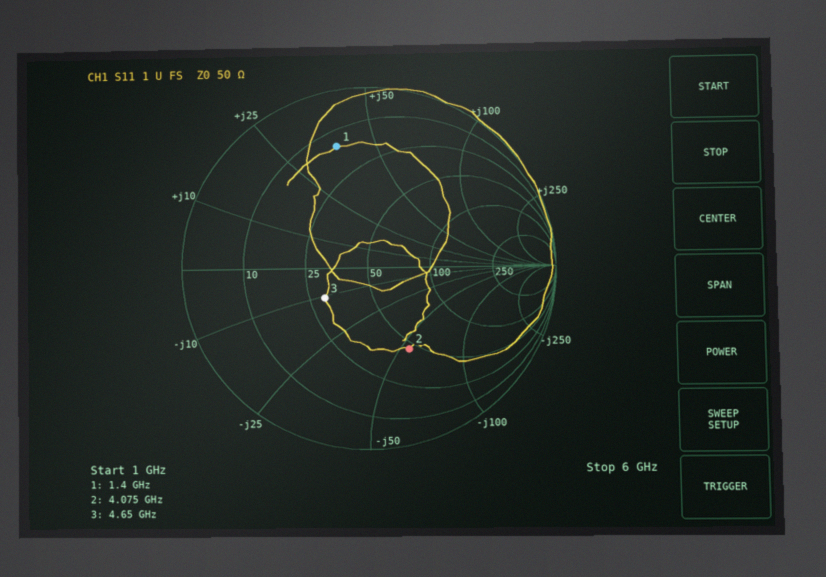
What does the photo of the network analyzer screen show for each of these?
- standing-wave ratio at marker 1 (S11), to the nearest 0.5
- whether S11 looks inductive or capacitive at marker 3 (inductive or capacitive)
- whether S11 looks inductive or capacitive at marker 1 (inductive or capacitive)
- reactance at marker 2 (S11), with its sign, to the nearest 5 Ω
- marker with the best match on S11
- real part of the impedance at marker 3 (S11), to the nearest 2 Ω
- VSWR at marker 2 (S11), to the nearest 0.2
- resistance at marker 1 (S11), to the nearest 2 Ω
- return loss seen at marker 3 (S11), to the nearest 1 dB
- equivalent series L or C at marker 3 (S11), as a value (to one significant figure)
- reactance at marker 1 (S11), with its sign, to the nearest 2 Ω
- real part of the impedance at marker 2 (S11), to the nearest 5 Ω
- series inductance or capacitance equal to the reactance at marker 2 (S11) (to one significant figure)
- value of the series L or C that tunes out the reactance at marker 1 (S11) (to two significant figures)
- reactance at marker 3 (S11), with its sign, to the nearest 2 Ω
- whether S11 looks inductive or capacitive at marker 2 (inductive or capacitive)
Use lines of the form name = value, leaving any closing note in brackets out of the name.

standing-wave ratio at marker 1 (S11), to the nearest 0.5 = 5.5
whether S11 looks inductive or capacitive at marker 3 = capacitive
whether S11 looks inductive or capacitive at marker 1 = inductive
reactance at marker 2 (S11), with its sign, to the nearest 5 Ω = -55 Ω
marker with the best match on S11 = marker 3
real part of the impedance at marker 3 (S11), to the nearest 2 Ω = 30 Ω
VSWR at marker 2 (S11), to the nearest 0.2 = 3.0
resistance at marker 1 (S11), to the nearest 2 Ω = 14 Ω
return loss seen at marker 3 (S11), to the nearest 1 dB = 11 dB
equivalent series L or C at marker 3 (S11), as a value = 3 pF
reactance at marker 1 (S11), with its sign, to the nearest 2 Ω = +38 Ω
real part of the impedance at marker 2 (S11), to the nearest 5 Ω = 45 Ω
series inductance or capacitance equal to the reactance at marker 2 (S11) = 700 fF
value of the series L or C that tunes out the reactance at marker 1 (S11) = 3.0 pF
reactance at marker 3 (S11), with its sign, to the nearest 2 Ω = -10 Ω
whether S11 looks inductive or capacitive at marker 2 = capacitive
